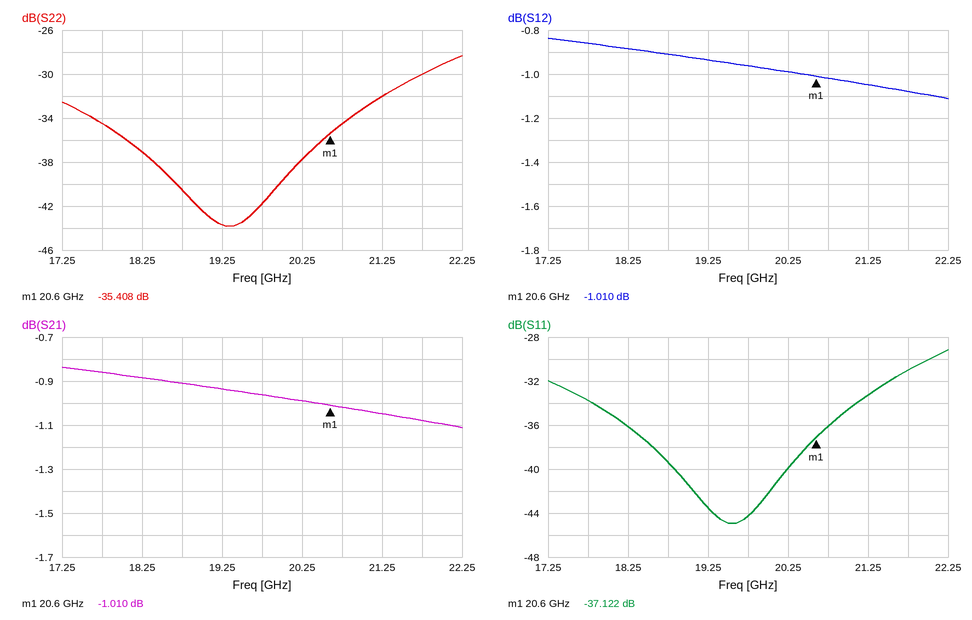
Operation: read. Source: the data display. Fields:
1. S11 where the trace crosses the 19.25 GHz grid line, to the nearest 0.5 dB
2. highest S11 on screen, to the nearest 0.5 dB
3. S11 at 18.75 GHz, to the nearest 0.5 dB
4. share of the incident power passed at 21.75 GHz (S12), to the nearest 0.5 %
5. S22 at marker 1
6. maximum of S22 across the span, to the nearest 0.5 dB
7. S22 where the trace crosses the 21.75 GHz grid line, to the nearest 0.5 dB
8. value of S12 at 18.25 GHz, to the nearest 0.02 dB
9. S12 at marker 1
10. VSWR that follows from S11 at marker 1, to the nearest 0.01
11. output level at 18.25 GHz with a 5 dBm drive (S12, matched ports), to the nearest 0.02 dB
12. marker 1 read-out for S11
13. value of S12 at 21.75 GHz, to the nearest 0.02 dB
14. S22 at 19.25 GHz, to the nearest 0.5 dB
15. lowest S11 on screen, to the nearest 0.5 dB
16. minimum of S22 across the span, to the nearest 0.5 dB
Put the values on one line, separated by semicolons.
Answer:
-43.5 dB; -29.0 dB; -39.5 dB; 78.0 %; -35.408 dB; -28.5 dB; -30.0 dB; -0.88 dB; -1.010 dB; 1.03; 4.12 dBm; -37.122 dB; -1.08 dB; -43.5 dB; -45.0 dB; -44.0 dB
